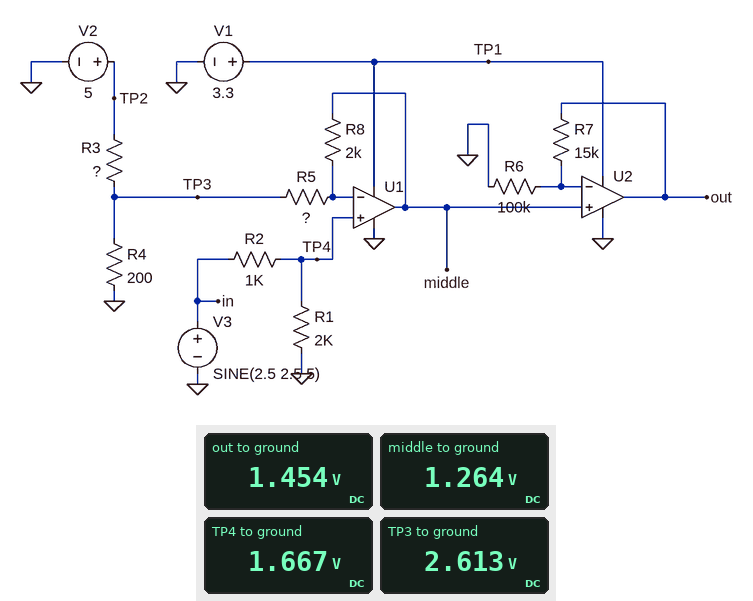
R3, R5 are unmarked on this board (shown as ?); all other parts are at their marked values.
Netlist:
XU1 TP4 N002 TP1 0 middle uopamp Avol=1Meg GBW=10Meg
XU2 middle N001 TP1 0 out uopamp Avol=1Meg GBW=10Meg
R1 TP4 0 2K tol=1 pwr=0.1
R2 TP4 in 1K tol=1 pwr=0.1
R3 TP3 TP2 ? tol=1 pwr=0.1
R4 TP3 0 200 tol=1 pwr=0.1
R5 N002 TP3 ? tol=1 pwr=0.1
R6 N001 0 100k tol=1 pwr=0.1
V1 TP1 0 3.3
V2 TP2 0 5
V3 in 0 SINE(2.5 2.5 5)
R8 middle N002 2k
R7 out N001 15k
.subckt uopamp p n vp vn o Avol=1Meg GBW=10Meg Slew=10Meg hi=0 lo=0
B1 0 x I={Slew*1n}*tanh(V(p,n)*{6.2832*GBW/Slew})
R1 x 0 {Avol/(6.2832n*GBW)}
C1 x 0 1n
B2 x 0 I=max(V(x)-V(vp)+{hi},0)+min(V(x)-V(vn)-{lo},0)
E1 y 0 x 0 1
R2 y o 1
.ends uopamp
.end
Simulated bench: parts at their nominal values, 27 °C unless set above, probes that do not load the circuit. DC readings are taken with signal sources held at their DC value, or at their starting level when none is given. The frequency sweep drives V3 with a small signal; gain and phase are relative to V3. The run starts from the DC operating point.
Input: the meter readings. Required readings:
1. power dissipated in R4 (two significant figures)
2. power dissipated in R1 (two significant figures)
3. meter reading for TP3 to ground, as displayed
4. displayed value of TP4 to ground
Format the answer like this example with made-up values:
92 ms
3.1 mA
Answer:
34 mW
1.4 mW
2.613 V
1.667 V
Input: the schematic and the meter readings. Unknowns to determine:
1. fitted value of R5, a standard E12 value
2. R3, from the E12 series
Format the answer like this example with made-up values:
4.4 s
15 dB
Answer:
4.7 kΩ
180 Ω
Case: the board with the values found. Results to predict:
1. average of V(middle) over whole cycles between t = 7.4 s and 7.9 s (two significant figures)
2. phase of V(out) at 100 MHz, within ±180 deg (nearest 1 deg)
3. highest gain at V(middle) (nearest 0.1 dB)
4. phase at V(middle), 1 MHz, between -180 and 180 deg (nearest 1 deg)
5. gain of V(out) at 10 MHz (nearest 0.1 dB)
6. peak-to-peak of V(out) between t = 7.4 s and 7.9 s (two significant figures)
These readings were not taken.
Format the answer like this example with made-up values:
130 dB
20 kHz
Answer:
1.5 V
-171 deg
-0.5 dB
-8 deg
-7.7 dB
3.3 V
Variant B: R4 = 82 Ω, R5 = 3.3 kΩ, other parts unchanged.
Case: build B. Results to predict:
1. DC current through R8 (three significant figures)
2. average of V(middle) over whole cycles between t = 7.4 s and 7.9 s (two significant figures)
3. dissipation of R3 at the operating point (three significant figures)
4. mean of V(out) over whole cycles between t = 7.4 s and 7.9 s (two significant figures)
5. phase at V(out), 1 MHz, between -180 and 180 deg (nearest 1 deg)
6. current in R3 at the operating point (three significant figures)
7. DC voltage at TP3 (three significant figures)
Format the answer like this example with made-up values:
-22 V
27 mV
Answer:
30.3 µA
1.7 V
65.5 mW
1.8 V
-16 deg
19.1 mA
1.57 V
